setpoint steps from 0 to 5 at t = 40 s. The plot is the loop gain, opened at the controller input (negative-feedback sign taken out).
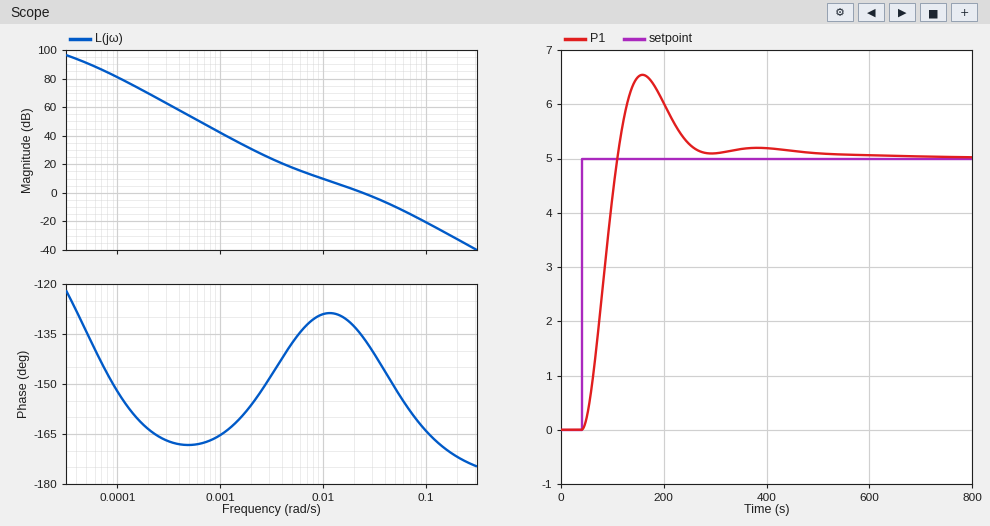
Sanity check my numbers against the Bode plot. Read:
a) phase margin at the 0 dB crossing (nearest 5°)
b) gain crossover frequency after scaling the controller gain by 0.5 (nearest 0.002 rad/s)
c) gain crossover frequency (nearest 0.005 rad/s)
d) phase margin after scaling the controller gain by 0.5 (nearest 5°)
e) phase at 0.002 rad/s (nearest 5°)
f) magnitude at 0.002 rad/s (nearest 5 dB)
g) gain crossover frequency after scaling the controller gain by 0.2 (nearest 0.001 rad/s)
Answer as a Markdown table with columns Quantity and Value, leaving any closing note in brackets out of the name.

| Quantity | Value |
|---|---|
| phase margin at the 0 dB crossing | 45° |
| gain crossover frequency after scaling the controller gain by 0.5 | 0.014 rad/s |
| gain crossover frequency | 0.025 rad/s |
| phase margin after scaling the controller gain by 0.5 | 50° |
| phase at 0.002 rad/s | -155° |
| magnitude at 0.002 rad/s | 30 dB |
| gain crossover frequency after scaling the controller gain by 0.2 | 0.007 rad/s |
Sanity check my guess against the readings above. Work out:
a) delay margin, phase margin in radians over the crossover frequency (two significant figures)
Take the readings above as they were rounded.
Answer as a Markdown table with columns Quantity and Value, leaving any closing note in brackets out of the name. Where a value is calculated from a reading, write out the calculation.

| Quantity | Value |
|---|---|
| delay margin, phase margin in radians over the crossover frequency | 45 × π / 180 / 0.025 = 31 s |
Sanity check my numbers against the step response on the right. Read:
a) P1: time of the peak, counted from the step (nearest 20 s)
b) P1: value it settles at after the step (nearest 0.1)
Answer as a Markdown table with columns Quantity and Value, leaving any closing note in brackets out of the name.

| Quantity | Value |
|---|---|
| P1: time of the peak, counted from the step | 120 s |
| P1: value it settles at after the step | 5.0 |
